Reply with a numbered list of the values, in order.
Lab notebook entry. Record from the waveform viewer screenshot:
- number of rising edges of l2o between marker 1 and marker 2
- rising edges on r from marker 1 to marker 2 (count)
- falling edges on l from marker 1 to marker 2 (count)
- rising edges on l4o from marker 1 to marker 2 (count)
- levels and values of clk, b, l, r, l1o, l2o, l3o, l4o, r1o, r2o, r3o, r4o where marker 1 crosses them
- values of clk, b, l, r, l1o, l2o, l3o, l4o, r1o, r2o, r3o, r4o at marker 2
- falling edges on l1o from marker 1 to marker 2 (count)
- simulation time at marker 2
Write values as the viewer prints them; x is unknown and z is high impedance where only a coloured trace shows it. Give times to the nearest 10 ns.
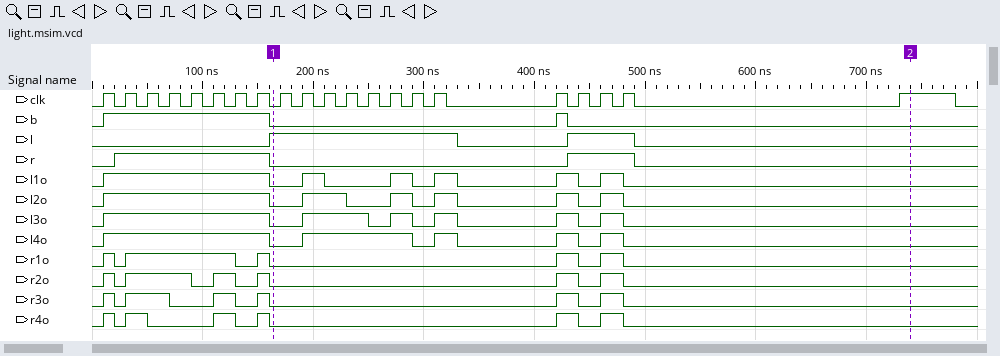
1. 5
2. 1
3. 2
4. 4
5. clk=0, b=0, l=1, r=0, l1o=0, l2o=0, l3o=0, l4o=0, r1o=0, r2o=0, r3o=0, r4o=0
6. clk=1, b=0, l=0, r=0, l1o=0, l2o=0, l3o=0, l4o=0, r1o=0, r2o=0, r3o=0, r4o=0
7. 5
8. 740 ns
